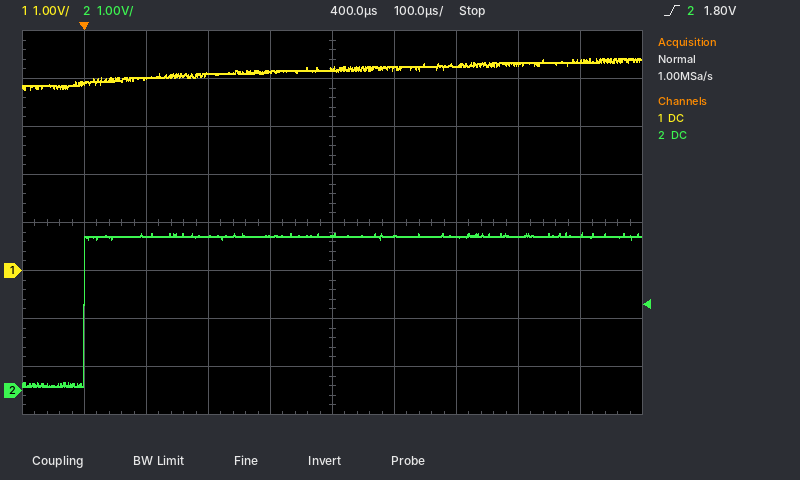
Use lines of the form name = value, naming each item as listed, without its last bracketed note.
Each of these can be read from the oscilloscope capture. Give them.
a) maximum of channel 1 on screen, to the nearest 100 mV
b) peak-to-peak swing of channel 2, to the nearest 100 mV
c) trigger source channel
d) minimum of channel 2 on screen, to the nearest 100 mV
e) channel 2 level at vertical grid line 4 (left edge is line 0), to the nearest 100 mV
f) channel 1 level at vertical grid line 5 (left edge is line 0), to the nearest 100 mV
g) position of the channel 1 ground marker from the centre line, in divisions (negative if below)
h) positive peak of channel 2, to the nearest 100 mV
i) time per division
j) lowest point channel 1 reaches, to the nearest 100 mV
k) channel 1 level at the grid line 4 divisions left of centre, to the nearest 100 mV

maximum of channel 1 on screen, to the nearest 100 mV = 4.4 V
peak-to-peak swing of channel 2, to the nearest 100 mV = 3.2 V
trigger source channel = channel 2
minimum of channel 2 on screen, to the nearest 100 mV = 100 mV
channel 2 level at vertical grid line 4 (left edge is line 0), to the nearest 100 mV = 3.2 V
channel 1 level at vertical grid line 5 (left edge is line 0), to the nearest 100 mV = 4.2 V
position of the channel 1 ground marker from the centre line, in divisions = -1.0 div
positive peak of channel 2, to the nearest 100 mV = 3.3 V
time per division = 100 µs
lowest point channel 1 reaches, to the nearest 100 mV = 3.8 V
channel 1 level at the grid line 4 divisions left of centre, to the nearest 100 mV = 3.9 V
